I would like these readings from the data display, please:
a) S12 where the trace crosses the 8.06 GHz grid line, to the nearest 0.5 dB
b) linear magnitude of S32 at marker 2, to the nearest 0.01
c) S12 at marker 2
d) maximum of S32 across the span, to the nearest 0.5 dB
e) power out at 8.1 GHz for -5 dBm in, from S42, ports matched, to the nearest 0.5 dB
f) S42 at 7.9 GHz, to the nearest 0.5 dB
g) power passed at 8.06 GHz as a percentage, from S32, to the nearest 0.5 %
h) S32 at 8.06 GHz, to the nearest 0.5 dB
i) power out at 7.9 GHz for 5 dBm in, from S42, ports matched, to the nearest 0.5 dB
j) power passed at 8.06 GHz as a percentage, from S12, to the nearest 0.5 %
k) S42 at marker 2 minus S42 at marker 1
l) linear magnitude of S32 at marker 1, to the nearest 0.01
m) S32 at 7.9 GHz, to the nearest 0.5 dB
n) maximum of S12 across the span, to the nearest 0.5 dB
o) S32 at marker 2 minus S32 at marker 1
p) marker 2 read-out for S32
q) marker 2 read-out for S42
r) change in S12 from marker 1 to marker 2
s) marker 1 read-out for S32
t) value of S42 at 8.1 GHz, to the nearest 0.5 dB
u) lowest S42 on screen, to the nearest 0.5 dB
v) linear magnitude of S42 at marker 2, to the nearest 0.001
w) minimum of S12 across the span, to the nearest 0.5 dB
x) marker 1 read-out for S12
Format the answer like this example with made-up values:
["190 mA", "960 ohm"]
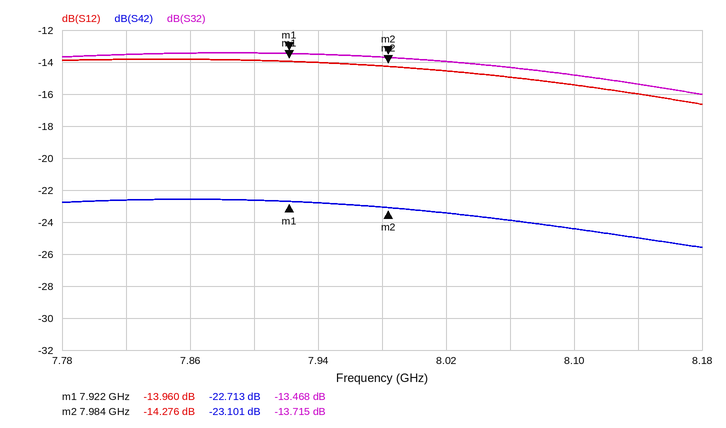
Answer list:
["-15.0 dB", "0.21", "-14.276 dB", "-13.5 dB", "-29.5 dBm", "-22.5 dB", "3.5 %", "-14.5 dB", "-17.5 dBm", "3.0 %", "-0.388 dB", "0.21", "-13.5 dB", "-14.0 dB", "-0.247 dB", "-13.715 dB", "-23.101 dB", "-0.316 dB", "-13.468 dB", "-24.5 dB", "-25.5 dB", "0.070", "-16.5 dB", "-13.960 dB"]
